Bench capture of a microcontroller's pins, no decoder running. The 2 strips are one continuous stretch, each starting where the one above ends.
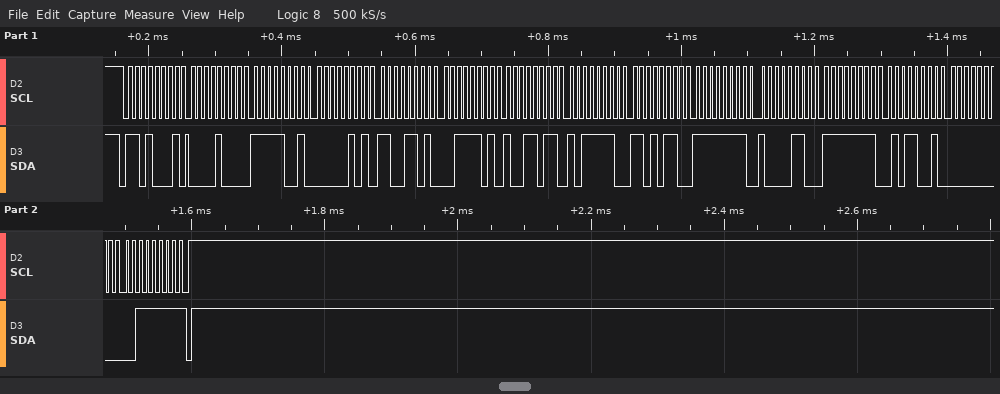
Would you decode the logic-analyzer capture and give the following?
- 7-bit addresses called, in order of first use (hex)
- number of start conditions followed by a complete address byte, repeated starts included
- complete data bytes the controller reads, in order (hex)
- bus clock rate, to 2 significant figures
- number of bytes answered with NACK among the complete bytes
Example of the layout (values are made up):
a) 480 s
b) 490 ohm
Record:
a) 0x68
b) 1
c) 08 F9 05 CD 3D 9B BE D6 FF 86 FF 59 00 3F
d) 100 kHz
e) 1
